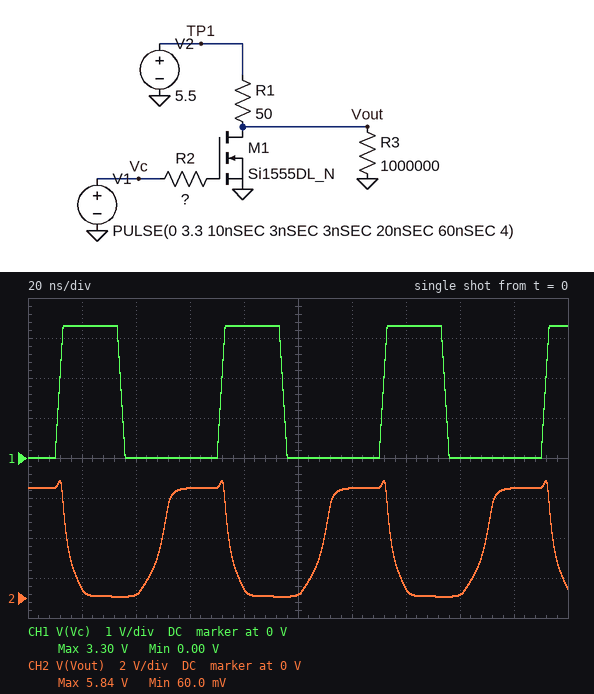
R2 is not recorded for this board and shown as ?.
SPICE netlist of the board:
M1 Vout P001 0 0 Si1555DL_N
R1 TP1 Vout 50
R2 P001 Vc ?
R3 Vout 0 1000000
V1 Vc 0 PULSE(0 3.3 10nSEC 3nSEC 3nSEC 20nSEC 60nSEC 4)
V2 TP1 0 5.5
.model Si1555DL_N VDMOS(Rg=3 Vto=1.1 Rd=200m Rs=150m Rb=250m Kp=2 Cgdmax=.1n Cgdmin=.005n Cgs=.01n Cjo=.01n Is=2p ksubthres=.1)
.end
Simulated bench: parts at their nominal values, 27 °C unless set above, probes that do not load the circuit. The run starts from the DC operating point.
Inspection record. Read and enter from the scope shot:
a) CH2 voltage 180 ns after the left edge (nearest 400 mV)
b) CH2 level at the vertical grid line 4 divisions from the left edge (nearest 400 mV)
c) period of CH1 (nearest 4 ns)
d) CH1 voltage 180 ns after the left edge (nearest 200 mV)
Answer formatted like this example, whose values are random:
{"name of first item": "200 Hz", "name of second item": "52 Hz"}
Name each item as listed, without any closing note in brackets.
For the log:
{"CH2 voltage 180 ns after the left edge": "5.6 V", "CH2 level at the vertical grid line 4 divisions from the left edge": "400 mV", "period of CH1": "60 ns", "CH1 voltage 180 ns after the left edge": "0 V"}
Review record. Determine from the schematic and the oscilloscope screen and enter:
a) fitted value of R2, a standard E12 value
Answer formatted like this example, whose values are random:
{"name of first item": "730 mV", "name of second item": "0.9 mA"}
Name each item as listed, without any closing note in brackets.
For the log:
{"fitted value of R2, a standard E12 value": "68 Ω"}
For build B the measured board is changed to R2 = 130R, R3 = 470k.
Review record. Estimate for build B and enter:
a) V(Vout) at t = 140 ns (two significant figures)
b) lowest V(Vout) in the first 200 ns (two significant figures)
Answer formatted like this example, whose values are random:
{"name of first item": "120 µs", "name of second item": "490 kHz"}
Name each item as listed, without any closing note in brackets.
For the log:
{"V(Vout) at t = 140 ns": "1.6 V", "lowest V(Vout) in the first 200 ns": "100 mV"}
